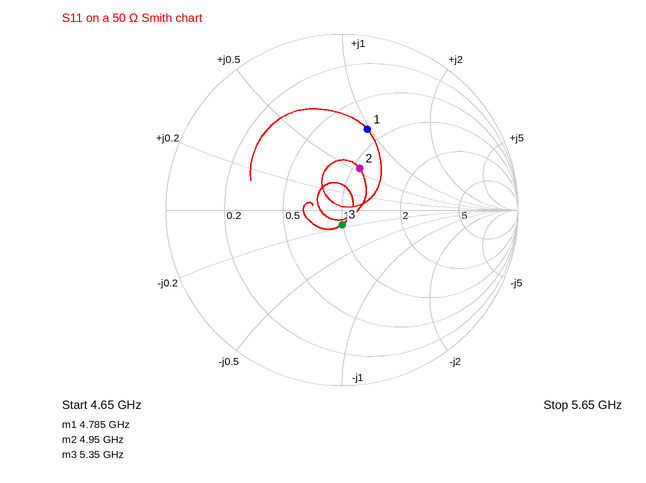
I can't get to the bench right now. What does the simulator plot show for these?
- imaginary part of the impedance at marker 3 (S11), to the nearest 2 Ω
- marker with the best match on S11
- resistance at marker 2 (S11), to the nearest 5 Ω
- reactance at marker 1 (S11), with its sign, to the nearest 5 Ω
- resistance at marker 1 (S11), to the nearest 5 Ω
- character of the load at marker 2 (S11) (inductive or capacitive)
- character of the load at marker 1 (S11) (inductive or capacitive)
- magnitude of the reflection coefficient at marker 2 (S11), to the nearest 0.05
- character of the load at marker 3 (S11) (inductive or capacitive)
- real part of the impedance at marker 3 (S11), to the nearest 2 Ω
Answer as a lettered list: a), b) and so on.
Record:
a) -8 Ω
b) marker 3
c) 55 Ω
d) +50 Ω
e) 40 Ω
f) inductive
g) inductive
h) 0.25
i) capacitive
j) 50 Ω
